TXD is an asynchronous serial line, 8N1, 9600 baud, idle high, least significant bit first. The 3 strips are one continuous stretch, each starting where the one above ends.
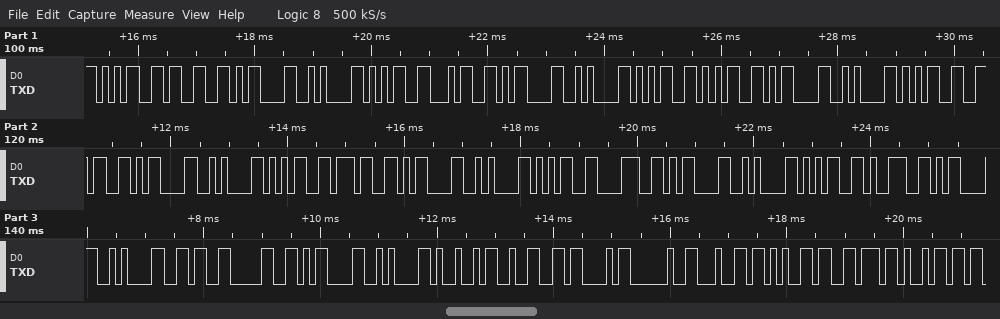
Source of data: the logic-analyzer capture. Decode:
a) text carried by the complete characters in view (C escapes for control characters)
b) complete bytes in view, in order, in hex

"53\r\n54\r\n55\r\n56\r\n57\r\n58\r\n59\r\n60\r\nI2C devi"
35 33 0D 0A 35 34 0D 0A 35 35 0D 0A 35 36 0D 0A 35 37 0D 0A 35 38 0D 0A 35 39 0D 0A 36 30 0D 0A 49 32 43 20 64 65 76 69
